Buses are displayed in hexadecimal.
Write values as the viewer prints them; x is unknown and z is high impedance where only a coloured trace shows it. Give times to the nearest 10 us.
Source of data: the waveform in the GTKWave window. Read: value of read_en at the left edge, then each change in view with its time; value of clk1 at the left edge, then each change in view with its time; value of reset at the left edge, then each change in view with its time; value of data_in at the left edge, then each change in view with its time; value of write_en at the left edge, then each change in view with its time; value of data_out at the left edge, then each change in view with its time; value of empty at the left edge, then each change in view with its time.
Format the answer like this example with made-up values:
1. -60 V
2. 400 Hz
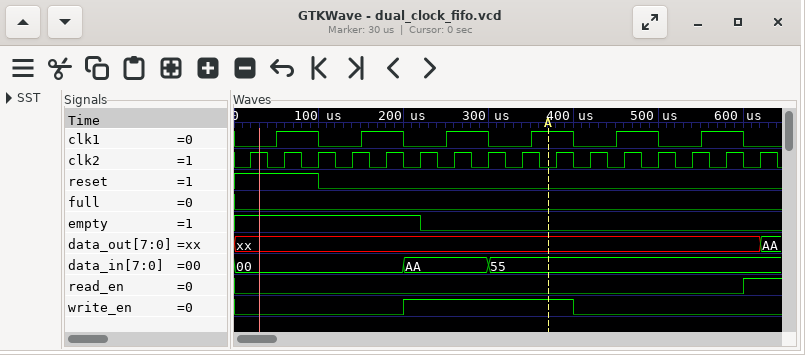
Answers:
1. 0, 1 at 600 us
2. 0, 1 at 50 us, 0 at 100 us, 1 at 150 us, 0 at 200 us, 1 at 250 us, 0 at 300 us, 1 at 350 us, 0 at 400 us, 1 at 450 us, 0 at 500 us, 1 at 550 us, 0 at 600 us
3. 1, 0 at 100 us
4. 00, AA at 200 us, 55 at 300 us
5. 0, 1 at 200 us, 0 at 400 us
6. xx, AA at 620 us
7. 1, 0 at 220 us
